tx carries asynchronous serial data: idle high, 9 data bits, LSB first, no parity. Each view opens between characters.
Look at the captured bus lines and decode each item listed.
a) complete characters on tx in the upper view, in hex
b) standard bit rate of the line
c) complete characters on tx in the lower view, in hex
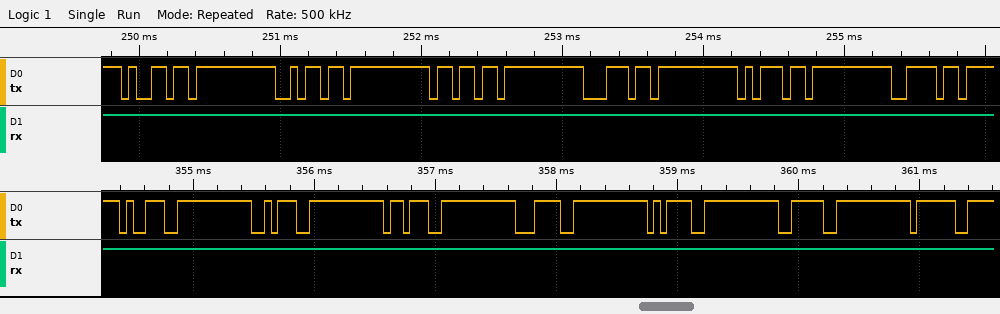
D9, DA, DB, DC, DD, DE
19200 baud
139, 13A, 13B, 13C, 13D, 13E, 13F
